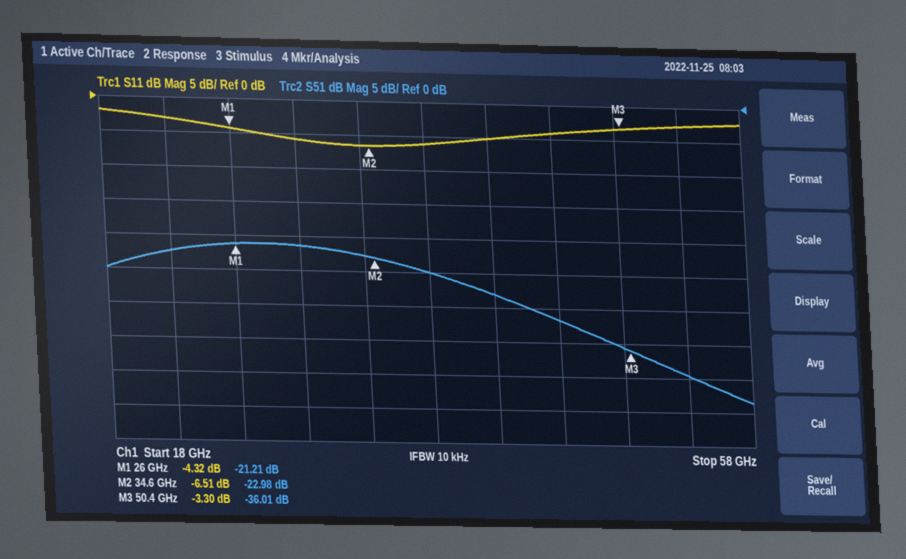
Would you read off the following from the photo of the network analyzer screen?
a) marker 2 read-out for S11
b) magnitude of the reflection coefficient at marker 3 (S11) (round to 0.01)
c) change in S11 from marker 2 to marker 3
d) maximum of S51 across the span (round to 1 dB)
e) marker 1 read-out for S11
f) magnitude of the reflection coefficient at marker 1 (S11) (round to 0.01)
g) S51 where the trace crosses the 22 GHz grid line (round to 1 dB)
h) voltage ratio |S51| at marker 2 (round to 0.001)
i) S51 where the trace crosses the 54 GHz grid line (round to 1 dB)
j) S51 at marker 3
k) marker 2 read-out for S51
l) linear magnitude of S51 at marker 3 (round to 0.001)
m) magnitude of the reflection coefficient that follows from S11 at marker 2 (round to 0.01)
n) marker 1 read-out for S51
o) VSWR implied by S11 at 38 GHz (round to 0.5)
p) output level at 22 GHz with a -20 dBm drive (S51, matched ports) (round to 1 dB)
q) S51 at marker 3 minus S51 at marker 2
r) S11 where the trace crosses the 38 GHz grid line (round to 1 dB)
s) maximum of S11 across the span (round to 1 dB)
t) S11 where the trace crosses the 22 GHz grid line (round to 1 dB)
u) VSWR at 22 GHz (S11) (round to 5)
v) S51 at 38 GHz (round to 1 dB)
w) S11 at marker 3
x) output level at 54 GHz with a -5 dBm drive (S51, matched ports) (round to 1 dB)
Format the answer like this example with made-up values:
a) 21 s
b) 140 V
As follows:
a) -6.51 dB
b) 0.68
c) 3.21 dB
d) -21 dB
e) -4.32 dB
f) 0.61
g) -22 dB
h) 0.071
i) -40 dB
j) -36.01 dB
k) -22.98 dB
l) 0.016
m) 0.47
n) -21.21 dB
o) 3.0
p) -42 dBm
q) -13.03 dB
r) -6 dB
s) -2 dB
t) -3 dB
u) 5
v) -25 dB
w) -3.30 dB
x) -45 dBm
